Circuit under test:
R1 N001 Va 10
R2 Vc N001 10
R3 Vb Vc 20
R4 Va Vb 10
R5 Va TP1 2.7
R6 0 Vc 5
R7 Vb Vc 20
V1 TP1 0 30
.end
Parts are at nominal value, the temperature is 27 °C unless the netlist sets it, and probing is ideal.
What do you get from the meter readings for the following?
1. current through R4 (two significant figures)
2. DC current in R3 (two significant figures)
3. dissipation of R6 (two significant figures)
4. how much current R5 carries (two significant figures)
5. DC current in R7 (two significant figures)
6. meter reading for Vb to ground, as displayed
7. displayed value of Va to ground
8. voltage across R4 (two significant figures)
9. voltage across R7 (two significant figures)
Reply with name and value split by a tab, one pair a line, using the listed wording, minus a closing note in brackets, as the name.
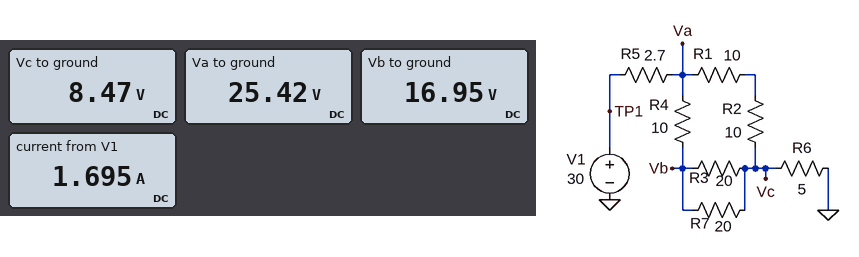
current through R4	850 mA
DC current in R3	420 mA
dissipation of R6	14 W
how much current R5 carries	1.7 A
DC current in R7	420 mA
meter reading for Vb to ground, as displayed	16.95 V
displayed value of Va to ground	25.42 V
voltage across R4	8.5 V
voltage across R7	8.5 V
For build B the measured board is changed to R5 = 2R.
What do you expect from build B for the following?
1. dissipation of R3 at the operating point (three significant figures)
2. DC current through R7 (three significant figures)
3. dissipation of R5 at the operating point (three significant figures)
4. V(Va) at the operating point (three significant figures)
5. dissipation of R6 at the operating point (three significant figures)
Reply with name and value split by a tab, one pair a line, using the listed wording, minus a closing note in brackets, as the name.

dissipation of R3 at the operating point	3.89 W
DC current through R7	441 mA
dissipation of R5 at the operating point	6.23 W
V(Va) at the operating point	26.5 V
dissipation of R6 at the operating point	15.6 W
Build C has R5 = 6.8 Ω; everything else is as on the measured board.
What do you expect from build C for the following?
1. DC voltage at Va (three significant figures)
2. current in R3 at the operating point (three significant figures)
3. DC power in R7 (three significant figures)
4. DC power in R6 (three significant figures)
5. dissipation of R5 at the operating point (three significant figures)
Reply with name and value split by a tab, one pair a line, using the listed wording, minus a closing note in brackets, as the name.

DC voltage at Va	20.6 V
current in R3 at the operating point	344 mA
DC power in R7	2.37 W
DC power in R6	9.47 W
dissipation of R5 at the operating point	12.9 W
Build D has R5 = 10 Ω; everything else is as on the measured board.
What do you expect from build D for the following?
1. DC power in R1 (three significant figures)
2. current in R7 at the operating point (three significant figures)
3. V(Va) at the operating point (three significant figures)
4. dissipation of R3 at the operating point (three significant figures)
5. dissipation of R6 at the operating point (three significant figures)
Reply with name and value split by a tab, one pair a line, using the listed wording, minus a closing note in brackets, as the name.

DC power in R1	3.60 W
current in R7 at the operating point	300 mA
V(Va) at the operating point	18.0 V
dissipation of R3 at the operating point	1.80 W
dissipation of R6 at the operating point	7.20 W
